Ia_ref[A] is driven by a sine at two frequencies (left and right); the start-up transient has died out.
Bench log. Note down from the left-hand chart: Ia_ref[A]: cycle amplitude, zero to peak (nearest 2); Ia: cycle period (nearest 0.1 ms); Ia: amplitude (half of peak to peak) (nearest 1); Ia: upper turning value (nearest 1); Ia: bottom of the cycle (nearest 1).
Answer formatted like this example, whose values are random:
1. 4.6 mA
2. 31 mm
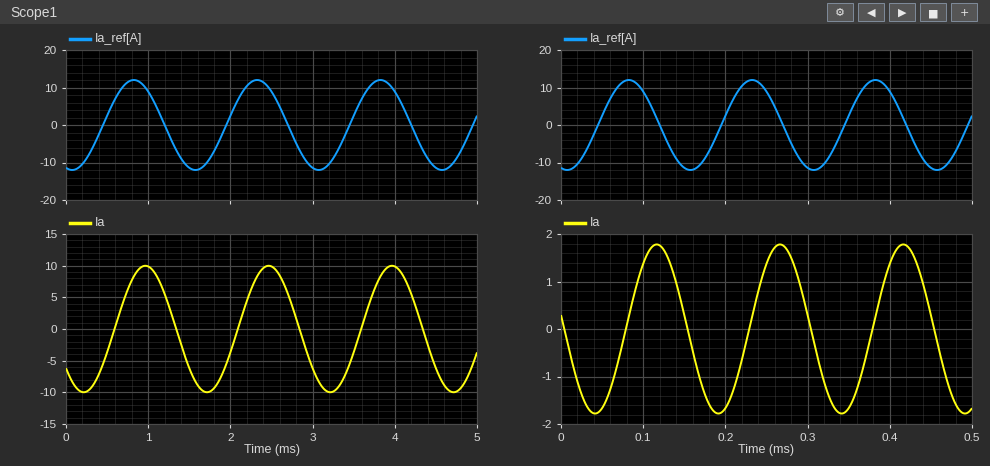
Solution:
1. 12
2. 1.5 ms
3. 10
4. 10
5. -10
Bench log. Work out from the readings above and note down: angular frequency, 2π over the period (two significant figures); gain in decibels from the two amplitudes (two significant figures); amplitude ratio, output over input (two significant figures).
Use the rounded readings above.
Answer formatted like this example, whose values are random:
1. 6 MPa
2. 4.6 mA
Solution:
1. 4.2 rad/ms
2. -1.6 dB
3. 0.83
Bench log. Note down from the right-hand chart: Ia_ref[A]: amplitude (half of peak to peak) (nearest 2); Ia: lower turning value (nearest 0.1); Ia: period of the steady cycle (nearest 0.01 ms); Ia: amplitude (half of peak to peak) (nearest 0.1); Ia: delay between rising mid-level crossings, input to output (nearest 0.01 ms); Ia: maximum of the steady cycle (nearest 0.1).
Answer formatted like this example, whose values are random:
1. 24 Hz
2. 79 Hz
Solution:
1. 12
2. -1.8
3. 0.15 ms
4. 1.8
5. 0.03 ms
6. 1.8
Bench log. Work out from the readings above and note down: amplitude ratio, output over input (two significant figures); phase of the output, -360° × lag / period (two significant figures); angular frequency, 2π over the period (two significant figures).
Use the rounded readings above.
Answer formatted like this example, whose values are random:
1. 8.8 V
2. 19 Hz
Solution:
1. 0.15
2. -72°
3. 42 rad/ms
